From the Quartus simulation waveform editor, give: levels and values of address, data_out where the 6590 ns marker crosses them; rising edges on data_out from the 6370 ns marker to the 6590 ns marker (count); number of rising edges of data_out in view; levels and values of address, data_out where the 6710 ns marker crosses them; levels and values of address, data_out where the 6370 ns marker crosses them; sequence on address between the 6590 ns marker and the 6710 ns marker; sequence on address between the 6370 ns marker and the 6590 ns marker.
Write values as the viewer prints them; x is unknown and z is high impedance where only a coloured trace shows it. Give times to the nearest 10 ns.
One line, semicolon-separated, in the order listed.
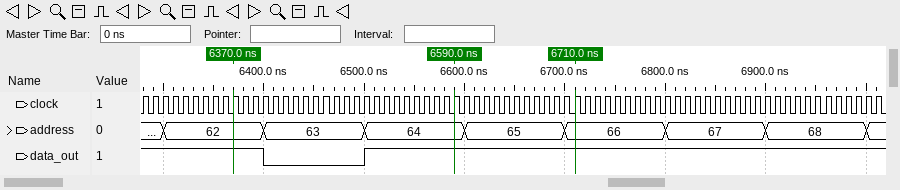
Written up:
address=64, data_out=1; 1; 1; address=66, data_out=1; address=62, data_out=1; 64, 65, 66; 62, 63, 64
